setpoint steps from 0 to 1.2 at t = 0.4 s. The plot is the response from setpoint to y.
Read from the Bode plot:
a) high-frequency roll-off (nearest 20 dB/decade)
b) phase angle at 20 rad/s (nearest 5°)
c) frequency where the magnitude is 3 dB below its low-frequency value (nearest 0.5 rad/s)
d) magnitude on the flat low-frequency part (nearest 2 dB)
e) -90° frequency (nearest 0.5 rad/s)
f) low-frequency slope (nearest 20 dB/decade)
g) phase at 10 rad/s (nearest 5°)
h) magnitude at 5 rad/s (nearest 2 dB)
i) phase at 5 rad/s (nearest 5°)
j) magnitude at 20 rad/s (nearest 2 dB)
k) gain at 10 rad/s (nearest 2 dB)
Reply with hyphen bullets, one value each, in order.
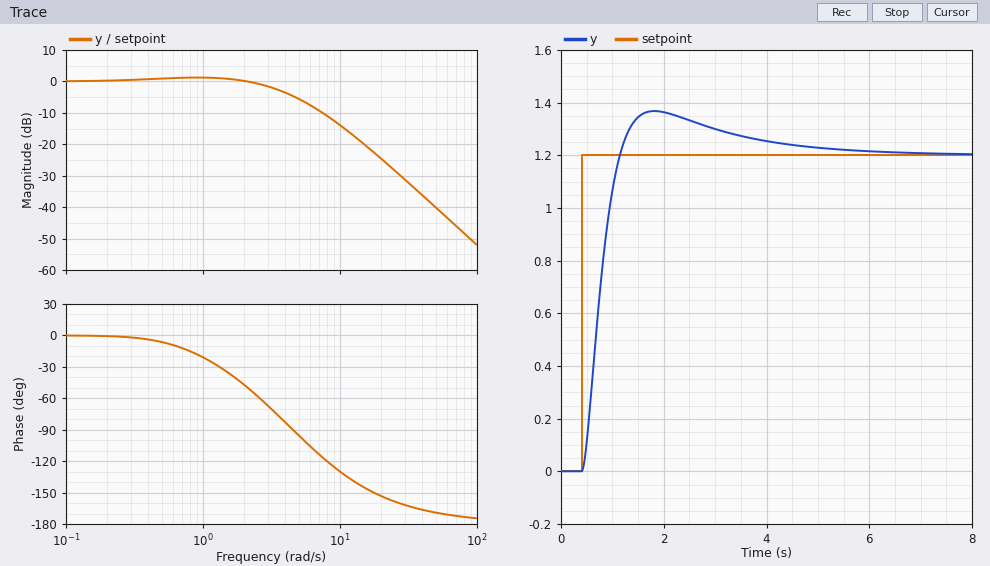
- -40 dB/decade
- -155°
- 3.5 rad/s
- 0 dB
- 4.5 rad/s
- 0 dB/decade
- -130°
- -6 dB
- -95°
- -24 dB
- -14 dB
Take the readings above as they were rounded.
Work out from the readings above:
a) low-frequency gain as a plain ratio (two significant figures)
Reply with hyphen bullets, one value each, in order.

- 1.0
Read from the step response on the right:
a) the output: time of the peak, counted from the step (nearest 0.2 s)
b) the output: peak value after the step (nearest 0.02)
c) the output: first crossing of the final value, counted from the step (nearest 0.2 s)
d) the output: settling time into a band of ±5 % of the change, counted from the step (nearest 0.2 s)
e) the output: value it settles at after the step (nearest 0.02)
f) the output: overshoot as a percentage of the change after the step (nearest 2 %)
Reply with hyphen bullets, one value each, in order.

- 1.4 s
- 1.36
- 0.8 s
- 3.4 s
- 1.20
- 14 %
